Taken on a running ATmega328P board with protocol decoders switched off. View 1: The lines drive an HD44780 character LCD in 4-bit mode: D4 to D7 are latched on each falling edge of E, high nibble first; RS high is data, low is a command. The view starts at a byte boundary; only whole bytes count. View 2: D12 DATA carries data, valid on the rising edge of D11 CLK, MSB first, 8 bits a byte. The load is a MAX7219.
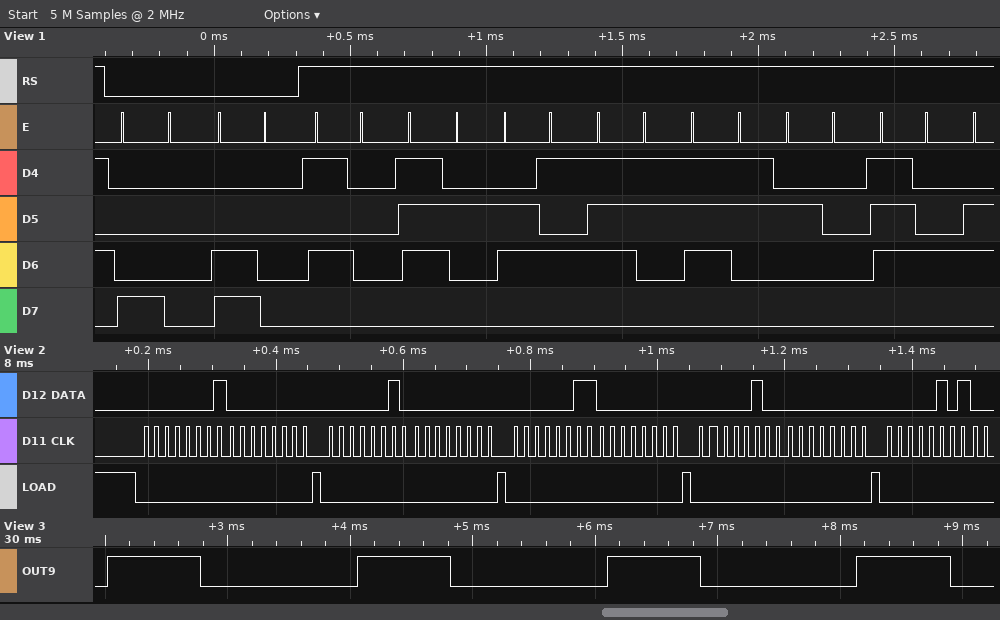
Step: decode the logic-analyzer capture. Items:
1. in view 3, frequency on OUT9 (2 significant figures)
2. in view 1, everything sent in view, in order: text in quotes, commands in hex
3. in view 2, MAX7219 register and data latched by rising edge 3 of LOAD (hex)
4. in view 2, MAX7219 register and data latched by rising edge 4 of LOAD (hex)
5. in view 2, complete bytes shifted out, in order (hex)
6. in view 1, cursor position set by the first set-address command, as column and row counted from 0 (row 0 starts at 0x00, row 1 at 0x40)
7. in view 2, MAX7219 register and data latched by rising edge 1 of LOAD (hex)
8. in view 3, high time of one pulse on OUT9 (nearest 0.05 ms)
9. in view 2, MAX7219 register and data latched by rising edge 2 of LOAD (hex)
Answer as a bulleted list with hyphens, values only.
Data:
- 490 Hz
- 0x80 0xC0 "Press t"
- register 0x3, data 0x00
- register 0x4, data 0x00
- 0x01 0x00 0x02 0x00 0x03 0x00 0x04 0x00 0x05
- column 0, row 0
- register 0x1, data 0x00
- 0.75 ms
- register 0x2, data 0x00
